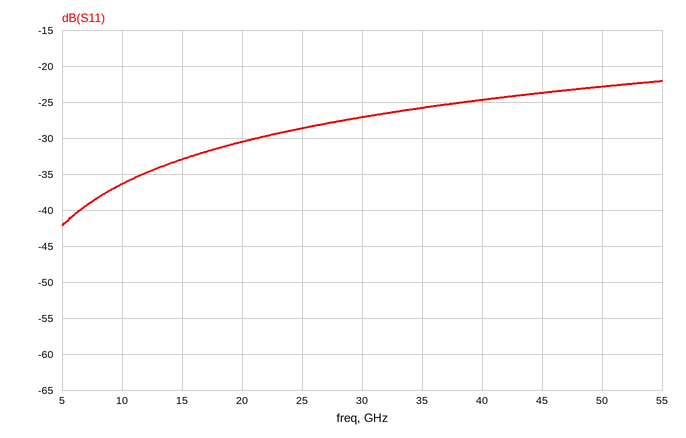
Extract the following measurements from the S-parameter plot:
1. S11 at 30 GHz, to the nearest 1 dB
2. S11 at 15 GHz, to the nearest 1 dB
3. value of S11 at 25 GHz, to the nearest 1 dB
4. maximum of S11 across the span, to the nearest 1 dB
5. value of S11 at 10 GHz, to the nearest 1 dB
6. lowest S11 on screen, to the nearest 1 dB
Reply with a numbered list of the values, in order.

1. -27 dB
2. -33 dB
3. -29 dB
4. -22 dB
5. -36 dB
6. -42 dB
